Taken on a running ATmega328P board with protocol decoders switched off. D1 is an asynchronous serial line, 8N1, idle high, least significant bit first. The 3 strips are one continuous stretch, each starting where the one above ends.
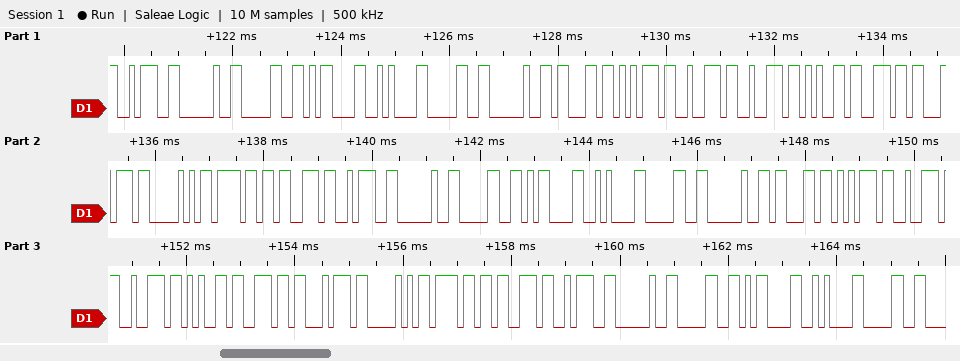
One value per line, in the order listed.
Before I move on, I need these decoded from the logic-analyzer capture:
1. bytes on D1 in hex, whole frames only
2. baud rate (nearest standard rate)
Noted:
3A 20 30 0D 0A 30 20 63 75 72 72 65 6E 74 50 6F 73 3A 20 30 0D 0A 30 20 63 75 72 72 65 6E 74 50 6F 73 3A 20 30 0D 0A 30
9600 baud
